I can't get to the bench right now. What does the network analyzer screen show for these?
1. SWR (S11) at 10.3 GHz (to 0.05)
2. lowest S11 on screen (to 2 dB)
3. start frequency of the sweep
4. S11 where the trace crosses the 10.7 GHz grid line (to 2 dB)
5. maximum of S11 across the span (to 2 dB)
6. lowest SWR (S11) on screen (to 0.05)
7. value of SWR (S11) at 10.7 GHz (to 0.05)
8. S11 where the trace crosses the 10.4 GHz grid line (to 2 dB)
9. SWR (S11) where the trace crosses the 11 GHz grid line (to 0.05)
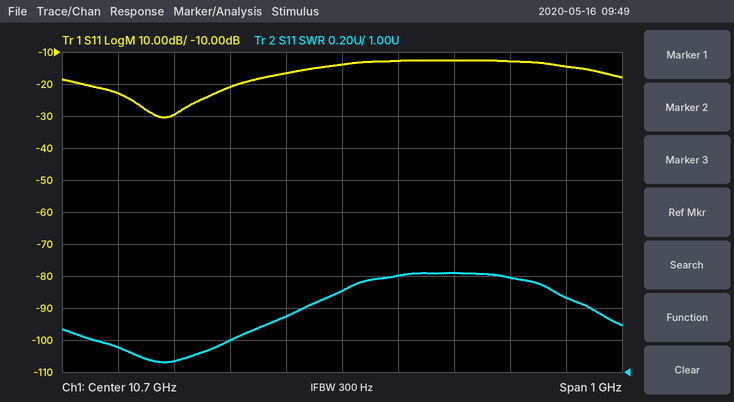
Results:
1.15
-30 dB
10.2 GHz
-14 dB
-12 dB
1.05
1.50
-30 dB
1.60
